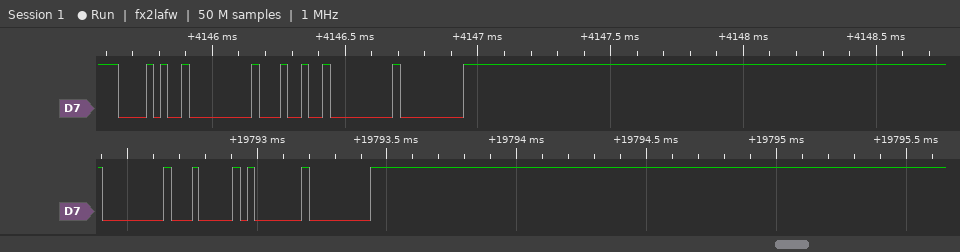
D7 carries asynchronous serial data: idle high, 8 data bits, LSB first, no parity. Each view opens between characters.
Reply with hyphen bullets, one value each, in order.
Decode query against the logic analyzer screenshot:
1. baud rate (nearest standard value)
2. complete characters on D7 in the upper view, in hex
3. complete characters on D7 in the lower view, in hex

- 38400 baud
- 28, 00, 24, 00, 00
- 00, 04, 01, 00
